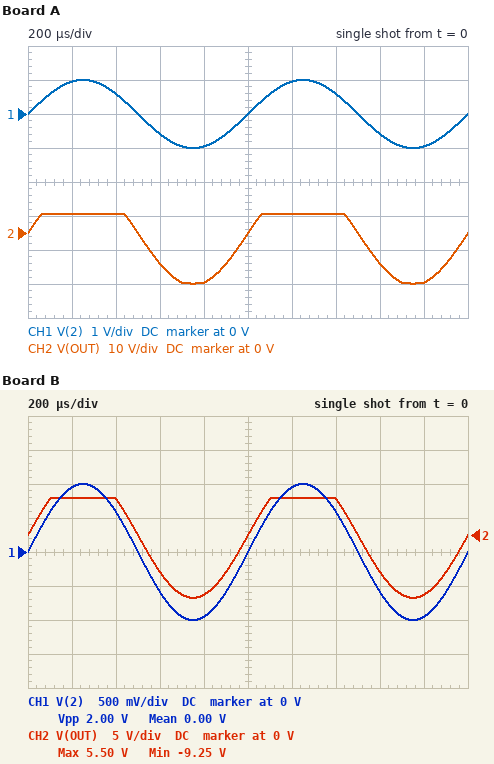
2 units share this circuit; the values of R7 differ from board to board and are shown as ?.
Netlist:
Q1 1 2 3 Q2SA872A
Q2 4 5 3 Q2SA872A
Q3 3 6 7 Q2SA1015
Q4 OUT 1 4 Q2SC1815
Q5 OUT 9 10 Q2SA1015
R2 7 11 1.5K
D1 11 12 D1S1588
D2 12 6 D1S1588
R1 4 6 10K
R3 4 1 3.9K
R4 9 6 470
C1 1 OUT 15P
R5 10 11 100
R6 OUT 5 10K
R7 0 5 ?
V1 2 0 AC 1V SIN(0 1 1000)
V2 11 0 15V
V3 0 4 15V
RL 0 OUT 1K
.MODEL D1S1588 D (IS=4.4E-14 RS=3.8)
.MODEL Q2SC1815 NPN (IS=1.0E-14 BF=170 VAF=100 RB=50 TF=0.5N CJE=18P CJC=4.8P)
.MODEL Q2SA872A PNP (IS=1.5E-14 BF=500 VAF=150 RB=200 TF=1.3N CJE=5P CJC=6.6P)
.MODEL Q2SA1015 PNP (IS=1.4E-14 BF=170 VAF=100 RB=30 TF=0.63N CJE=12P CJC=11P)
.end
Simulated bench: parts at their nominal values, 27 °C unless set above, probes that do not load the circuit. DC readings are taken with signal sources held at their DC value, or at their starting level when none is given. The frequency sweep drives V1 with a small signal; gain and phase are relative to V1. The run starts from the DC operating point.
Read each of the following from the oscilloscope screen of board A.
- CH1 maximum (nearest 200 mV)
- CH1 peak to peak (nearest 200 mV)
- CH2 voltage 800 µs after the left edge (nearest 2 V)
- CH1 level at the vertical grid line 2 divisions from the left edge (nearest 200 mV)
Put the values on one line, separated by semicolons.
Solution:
1.0 V; 2.0 V; -14 V; 600 mV
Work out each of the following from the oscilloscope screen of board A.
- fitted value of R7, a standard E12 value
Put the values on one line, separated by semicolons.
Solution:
680 Ω
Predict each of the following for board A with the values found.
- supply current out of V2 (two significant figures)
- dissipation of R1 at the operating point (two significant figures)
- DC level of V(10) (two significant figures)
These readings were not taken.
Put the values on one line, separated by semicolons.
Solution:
9.3 mA; 82 mW; 14 V
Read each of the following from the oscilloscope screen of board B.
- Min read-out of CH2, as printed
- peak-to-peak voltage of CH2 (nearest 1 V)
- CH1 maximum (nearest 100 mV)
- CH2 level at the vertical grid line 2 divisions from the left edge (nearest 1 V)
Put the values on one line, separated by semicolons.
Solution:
-9.25 V; 15 V; 1.0 V; 5 V
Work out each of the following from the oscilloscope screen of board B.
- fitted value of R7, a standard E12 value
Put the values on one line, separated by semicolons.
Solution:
1.2 kΩ
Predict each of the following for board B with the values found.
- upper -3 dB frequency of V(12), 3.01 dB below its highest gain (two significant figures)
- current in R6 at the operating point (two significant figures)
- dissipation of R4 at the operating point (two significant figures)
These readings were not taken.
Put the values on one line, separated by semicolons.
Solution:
2.6 GHz; 3.5 µA; 450 nW
